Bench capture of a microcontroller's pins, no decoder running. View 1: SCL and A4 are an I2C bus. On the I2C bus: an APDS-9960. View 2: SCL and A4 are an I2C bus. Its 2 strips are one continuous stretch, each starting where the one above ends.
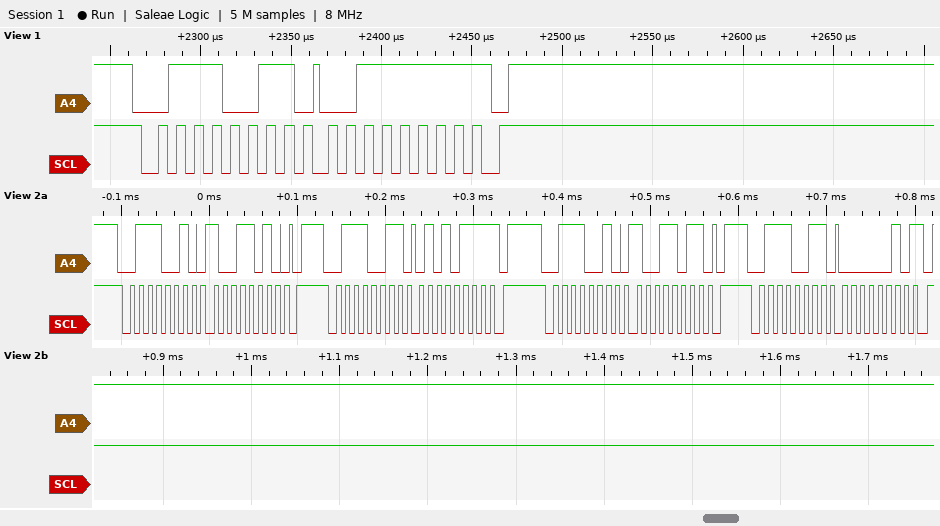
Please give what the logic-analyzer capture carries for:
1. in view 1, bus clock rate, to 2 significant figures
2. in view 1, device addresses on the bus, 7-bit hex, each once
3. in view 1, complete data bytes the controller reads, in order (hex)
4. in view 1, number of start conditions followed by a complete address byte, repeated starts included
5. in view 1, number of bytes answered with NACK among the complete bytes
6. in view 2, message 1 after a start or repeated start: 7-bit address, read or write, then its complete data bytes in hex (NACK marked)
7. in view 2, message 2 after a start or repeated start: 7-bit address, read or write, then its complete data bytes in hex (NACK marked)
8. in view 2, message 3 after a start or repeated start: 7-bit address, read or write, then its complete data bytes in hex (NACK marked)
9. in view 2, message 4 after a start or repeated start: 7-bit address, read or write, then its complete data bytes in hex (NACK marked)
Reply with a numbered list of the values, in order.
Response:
1. 100 kHz
2. 0x39
3. 3F
4. 1
5. 1
6. 0x39 write: 9A
7. 0x39 read: 57 NACK
8. 0x39 write: 9B
9. 0x39 read: 02 NACK
